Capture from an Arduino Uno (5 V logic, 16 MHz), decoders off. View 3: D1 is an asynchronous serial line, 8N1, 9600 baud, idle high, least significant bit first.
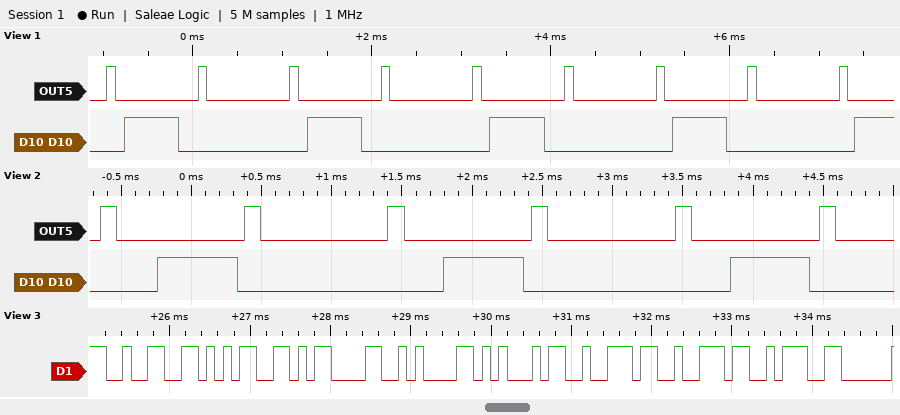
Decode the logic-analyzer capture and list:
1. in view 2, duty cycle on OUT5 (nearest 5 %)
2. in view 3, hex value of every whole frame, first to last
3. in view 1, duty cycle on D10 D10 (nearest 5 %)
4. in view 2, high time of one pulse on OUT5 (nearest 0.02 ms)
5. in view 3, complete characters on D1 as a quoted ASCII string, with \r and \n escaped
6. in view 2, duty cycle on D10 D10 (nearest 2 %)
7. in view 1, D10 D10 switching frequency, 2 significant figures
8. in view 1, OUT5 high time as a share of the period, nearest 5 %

10 %
32 35 0D 0A 45 72 72 3A
30 %
0.12 ms
"25\r\nErr:"
28 %
490 Hz
10 %
